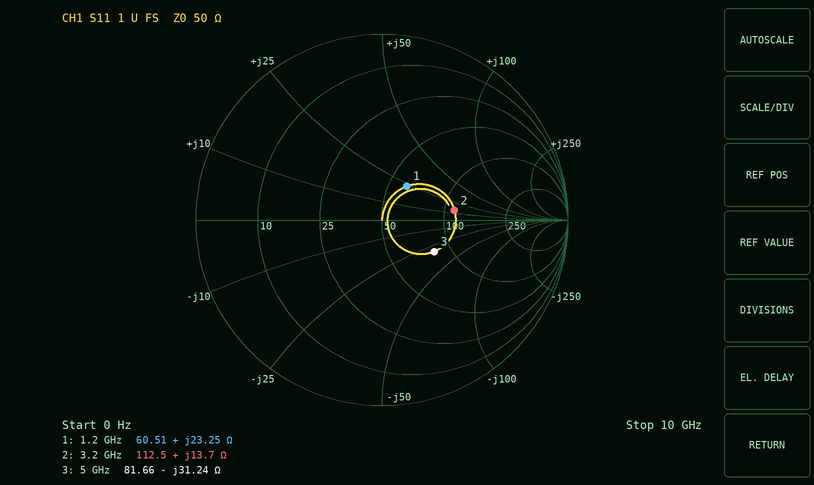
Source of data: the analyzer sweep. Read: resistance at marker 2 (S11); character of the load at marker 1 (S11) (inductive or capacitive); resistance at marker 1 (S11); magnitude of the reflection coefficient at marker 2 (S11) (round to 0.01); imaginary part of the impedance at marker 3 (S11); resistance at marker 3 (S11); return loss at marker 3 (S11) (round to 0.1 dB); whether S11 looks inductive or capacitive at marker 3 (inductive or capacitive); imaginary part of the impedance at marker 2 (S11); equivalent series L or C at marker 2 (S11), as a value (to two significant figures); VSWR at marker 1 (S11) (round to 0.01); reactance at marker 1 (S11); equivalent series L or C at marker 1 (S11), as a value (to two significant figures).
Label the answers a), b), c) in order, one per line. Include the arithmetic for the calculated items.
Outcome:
a) 112.5 Ω
b) inductive
c) 60.51 Ω
d) 0.39
e) -31.24 Ω
f) 81.66 Ω
g) 9.7 dB
h) capacitive
i) +13.7 Ω
j) L = 13.7 Ω/(2π × 3.2 GHz) ≈ 681 pH, so 680 pH to two significant figures
k) 1.58
l) +23.25 Ω
m) L = 23.25 Ω/(2π × 1.2 GHz) ≈ 3.1 nH
